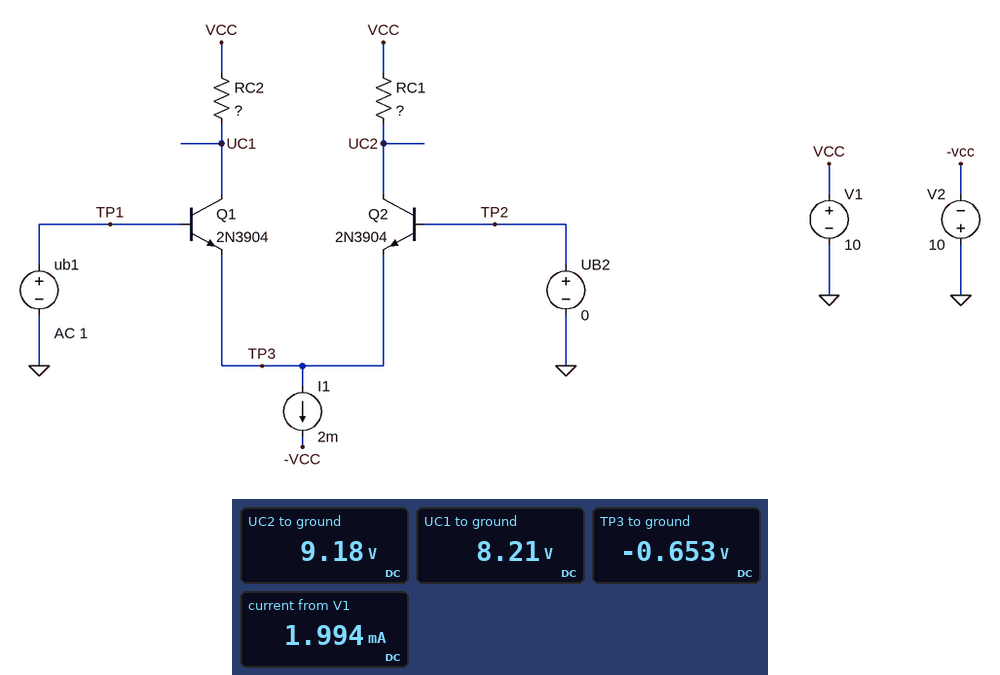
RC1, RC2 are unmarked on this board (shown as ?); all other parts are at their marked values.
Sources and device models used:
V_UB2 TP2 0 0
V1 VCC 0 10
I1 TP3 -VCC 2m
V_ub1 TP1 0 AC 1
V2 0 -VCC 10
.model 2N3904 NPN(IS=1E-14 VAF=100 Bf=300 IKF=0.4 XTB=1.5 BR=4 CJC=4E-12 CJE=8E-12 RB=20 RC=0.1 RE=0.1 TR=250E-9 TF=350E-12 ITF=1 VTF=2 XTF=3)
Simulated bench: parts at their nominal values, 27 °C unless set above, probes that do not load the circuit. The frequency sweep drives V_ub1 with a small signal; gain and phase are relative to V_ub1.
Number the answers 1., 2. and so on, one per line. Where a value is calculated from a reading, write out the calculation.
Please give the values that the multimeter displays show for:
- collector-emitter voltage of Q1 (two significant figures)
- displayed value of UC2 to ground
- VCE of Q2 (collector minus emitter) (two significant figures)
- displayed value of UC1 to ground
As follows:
1. 8.21 V - (-653 mV) = 8.9 V
2. 9.18 V
3. 9.18 V - (-653 mV) = 9.8 V
4. 8.21 V
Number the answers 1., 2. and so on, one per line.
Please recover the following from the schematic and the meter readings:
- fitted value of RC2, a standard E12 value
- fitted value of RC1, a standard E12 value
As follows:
1. 1.8 kΩ
2. 820 Ω
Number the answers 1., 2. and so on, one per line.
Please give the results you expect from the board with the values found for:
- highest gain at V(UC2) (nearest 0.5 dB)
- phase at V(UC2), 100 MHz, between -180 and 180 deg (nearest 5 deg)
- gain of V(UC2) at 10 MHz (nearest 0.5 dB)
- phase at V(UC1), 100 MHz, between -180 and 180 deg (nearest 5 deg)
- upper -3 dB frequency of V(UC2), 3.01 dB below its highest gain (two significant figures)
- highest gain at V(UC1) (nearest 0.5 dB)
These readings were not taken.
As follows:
1. 24.0 dB
2. -65 deg
3. 23.5 dB
4. 90 deg
5. 45 MHz
6. 30.5 dB
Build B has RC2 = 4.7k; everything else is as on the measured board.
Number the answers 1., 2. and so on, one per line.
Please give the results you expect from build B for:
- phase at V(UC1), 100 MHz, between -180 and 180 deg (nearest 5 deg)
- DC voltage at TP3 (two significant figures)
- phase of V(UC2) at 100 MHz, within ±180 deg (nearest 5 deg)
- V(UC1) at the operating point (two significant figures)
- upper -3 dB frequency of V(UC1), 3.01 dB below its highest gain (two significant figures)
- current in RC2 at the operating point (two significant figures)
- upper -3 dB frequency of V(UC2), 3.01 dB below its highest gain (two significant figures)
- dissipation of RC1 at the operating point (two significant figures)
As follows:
1. 75 deg
2. -650 mV
3. -60 deg
4. 5.4 V
5. 12 MHz
6. 980 µA
7. 33 MHz
8. 840 µW
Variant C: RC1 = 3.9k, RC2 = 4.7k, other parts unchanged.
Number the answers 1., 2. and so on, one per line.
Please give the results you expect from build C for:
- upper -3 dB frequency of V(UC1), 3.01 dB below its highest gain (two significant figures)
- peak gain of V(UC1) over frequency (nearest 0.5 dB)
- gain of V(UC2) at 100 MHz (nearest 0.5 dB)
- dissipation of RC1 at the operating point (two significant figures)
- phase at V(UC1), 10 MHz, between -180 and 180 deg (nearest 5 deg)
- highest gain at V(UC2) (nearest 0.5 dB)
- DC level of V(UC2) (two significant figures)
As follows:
1. 10 MHz
2. 38.5 dB
3. 18.5 dB
4. 3.9 mW
5. 135 deg
6. 37.0 dB
7. 6.1 V
